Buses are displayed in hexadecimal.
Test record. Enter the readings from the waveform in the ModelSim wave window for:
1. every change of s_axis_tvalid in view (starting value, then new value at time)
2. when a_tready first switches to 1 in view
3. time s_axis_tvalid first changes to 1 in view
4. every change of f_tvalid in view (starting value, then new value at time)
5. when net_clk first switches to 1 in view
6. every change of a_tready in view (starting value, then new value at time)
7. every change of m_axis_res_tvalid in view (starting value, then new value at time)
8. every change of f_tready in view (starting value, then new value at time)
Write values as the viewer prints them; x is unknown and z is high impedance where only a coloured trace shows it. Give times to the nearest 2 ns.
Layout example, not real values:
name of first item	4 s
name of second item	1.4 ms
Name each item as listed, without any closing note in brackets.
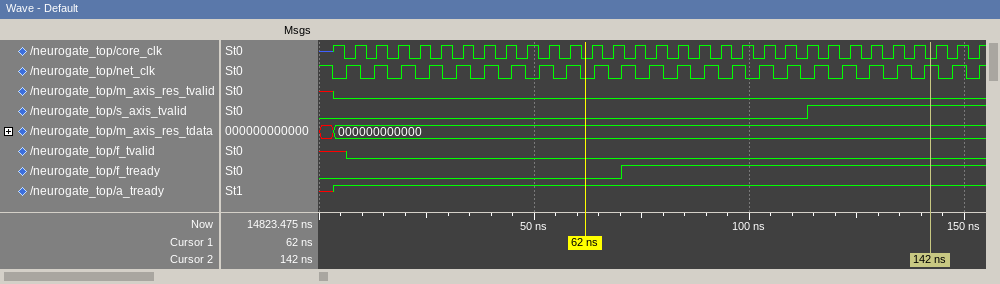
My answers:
every change of s_axis_tvalid in view	0, 1 at 114 ns
when a_tready first switches to 1 in view	4 ns
time s_axis_tvalid first changes to 1 in view	114 ns
every change of f_tvalid in view	x, 0 at 6 ns
when net_clk first switches to 1 in view	6 ns
every change of a_tready in view	x, 1 at 4 ns
every change of m_axis_res_tvalid in view	x, 0 at 4 ns
every change of f_tready in view	0, 1 at 70 ns
